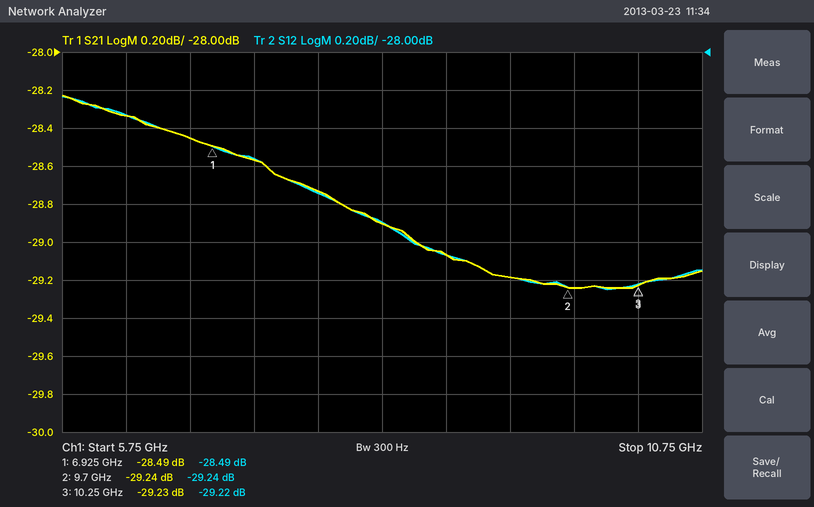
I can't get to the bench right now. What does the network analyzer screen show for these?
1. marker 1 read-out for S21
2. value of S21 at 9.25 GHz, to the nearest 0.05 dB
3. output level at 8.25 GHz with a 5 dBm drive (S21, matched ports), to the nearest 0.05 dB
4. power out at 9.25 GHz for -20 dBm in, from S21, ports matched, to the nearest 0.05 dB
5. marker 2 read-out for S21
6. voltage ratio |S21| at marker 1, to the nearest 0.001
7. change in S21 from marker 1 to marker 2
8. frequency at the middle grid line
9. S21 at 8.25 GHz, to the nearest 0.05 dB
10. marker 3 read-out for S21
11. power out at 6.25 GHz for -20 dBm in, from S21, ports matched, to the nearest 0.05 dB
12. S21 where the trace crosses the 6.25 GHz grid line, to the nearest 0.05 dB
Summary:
-28.49 dB
-29.20 dB
-23.90 dBm
-49.20 dBm
-29.24 dB
0.038
-0.75 dB
8.25 GHz
-28.90 dB
-29.23 dB
-48.35 dBm
-28.35 dB
